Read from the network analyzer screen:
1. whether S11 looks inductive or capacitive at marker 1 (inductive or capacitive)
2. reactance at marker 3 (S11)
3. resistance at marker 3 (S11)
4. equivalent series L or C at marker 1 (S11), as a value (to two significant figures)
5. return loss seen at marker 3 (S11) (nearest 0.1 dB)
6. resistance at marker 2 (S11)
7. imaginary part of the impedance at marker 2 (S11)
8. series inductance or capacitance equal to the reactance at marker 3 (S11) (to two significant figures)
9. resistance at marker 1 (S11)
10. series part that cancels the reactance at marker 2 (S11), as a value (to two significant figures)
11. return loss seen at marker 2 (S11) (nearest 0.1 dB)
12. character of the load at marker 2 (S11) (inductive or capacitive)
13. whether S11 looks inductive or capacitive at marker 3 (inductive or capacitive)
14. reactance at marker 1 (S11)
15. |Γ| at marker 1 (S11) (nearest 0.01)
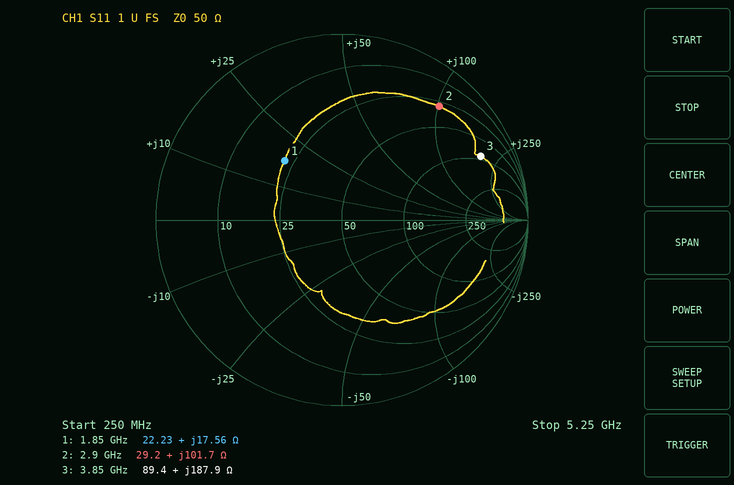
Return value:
inductive
+187.9 Ω
89.4 Ω
1.5 nH
1.7 dB
29.2 Ω
+101.7 Ω
7.8 nH
22.23 Ω
540 fF
1.9 dB
inductive
inductive
+17.56 Ω
0.44
